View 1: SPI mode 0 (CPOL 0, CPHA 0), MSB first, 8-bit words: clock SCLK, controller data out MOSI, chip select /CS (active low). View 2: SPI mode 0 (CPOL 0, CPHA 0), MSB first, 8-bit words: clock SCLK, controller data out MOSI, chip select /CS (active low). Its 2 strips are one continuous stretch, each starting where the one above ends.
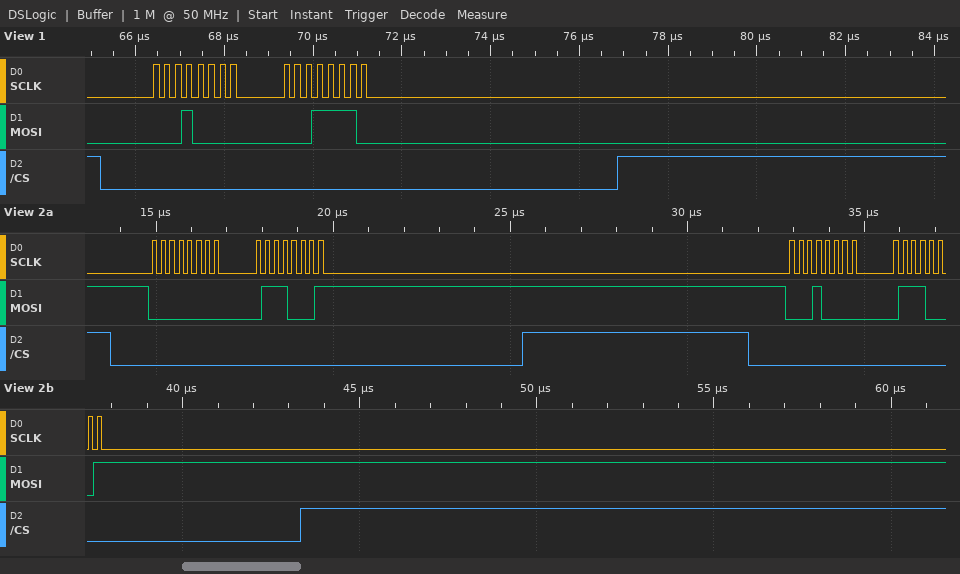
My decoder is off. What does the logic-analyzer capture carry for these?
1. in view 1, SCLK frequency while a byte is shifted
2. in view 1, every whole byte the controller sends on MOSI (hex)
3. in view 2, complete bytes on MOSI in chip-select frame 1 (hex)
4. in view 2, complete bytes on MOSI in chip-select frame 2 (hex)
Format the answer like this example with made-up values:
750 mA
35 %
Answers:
4 MHz
10 1E
0x00 0x71
0x10 0x71
